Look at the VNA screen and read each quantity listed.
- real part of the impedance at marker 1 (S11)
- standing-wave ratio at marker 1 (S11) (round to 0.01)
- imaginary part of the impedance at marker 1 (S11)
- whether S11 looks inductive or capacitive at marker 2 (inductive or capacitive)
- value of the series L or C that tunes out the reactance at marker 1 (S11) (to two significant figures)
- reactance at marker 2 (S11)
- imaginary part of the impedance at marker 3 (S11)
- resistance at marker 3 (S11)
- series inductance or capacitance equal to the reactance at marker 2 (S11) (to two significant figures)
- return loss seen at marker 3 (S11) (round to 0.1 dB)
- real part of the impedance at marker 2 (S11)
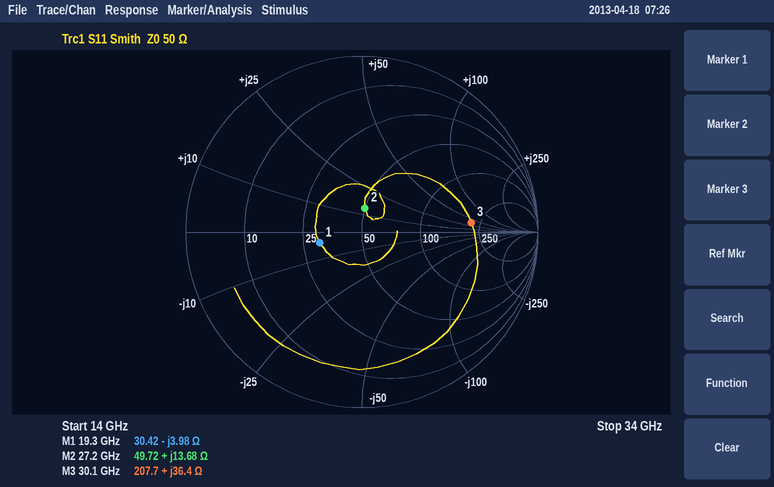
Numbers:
30.42 Ω
1.66
-3.98 Ω
inductive
33 pH
+13.68 Ω
+36.4 Ω
207.7 Ω
80 pH
4.1 dB
49.72 Ω
